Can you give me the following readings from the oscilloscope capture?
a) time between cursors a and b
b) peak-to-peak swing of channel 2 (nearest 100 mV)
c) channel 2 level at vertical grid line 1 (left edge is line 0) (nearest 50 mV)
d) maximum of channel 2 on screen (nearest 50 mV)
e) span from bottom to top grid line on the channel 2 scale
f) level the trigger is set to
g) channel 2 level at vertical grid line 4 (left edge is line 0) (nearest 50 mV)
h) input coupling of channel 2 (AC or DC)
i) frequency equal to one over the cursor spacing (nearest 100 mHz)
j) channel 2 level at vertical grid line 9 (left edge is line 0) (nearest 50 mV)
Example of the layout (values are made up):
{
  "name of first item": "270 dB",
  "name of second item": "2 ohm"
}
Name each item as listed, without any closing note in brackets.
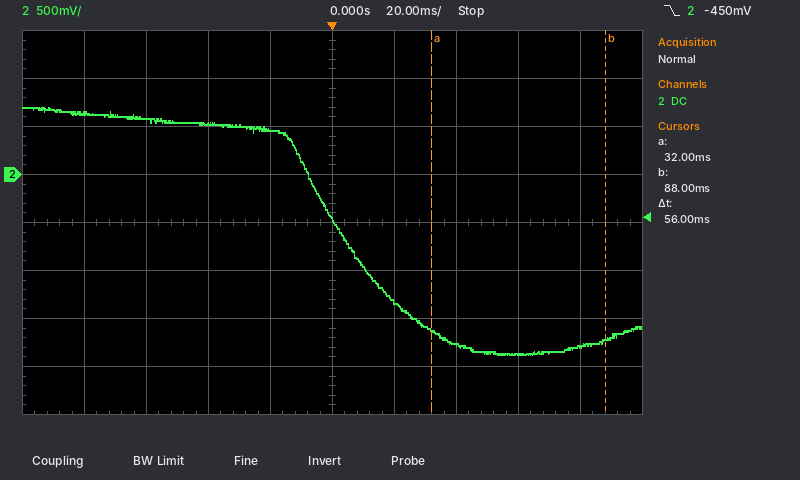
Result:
{
  "time between cursors a and b": "56 ms",
  "peak-to-peak swing of channel 2": "2.60 V",
  "channel 2 level at vertical grid line 1 (left edge is line 0)": "650 mV",
  "maximum of channel 2 on screen": "700 mV",
  "span from bottom to top grid line on the channel 2 scale": "4 V",
  "level the trigger is set to": "-450 mV",
  "channel 2 level at vertical grid line 4 (left edge is line 0)": "450 mV",
  "input coupling of channel 2": "DC",
  "frequency equal to one over the cursor spacing": "17.9 Hz",
  "channel 2 level at vertical grid line 9 (left edge is line 0)": "-1.80 V"
}
